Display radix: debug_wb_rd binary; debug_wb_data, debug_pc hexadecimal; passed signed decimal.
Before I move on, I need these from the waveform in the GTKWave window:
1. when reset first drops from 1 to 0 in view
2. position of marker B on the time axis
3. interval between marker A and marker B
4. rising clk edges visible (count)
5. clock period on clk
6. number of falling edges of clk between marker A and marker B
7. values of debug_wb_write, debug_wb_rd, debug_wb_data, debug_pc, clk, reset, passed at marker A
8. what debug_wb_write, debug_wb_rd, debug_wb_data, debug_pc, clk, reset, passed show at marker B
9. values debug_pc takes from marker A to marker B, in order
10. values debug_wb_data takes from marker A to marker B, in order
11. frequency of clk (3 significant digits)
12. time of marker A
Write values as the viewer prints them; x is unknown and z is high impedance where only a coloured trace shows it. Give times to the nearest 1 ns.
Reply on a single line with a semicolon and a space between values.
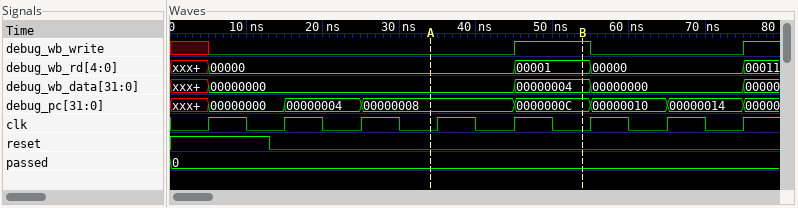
13 ns; 54 ns; 20 ns; 8; 10 ns; 2; debug_wb_write=0, debug_wb_rd=00000, debug_wb_data=00000000, debug_pc=00000008, clk=0, reset=0, passed=0; debug_wb_write=1, debug_wb_rd=00001, debug_wb_data=00000004, debug_pc=0000000C, clk=0, reset=0, passed=0; 00000008, 0000000C; 00000000, 00000004; 100 MHz; 34 ns
